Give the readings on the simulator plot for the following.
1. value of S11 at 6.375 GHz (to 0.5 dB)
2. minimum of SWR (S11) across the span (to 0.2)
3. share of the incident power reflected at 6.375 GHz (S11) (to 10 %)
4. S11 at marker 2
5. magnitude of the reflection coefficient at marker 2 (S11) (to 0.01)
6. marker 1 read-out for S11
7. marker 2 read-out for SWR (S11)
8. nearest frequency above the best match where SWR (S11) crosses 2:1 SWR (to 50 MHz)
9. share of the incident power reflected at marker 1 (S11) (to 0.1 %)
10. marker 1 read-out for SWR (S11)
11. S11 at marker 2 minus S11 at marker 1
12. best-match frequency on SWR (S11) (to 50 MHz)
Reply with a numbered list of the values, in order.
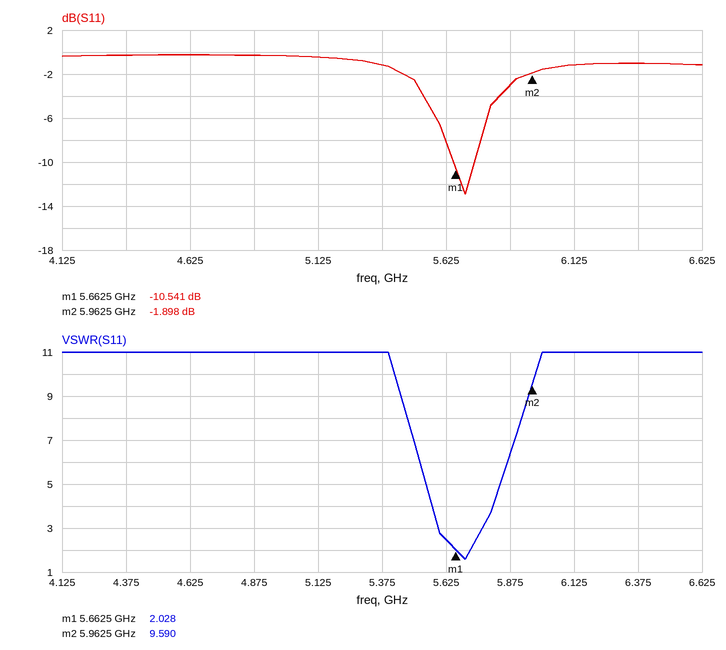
1. -1.0 dB
2. 1.6
3. 80 %
4. -1.898 dB
5. 0.80
6. -10.541 dB
7. 9.590
8. 5.70 GHz
9. 8.8 %
10. 2.028
11. 8.643 dB
12. 5.70 GHz
